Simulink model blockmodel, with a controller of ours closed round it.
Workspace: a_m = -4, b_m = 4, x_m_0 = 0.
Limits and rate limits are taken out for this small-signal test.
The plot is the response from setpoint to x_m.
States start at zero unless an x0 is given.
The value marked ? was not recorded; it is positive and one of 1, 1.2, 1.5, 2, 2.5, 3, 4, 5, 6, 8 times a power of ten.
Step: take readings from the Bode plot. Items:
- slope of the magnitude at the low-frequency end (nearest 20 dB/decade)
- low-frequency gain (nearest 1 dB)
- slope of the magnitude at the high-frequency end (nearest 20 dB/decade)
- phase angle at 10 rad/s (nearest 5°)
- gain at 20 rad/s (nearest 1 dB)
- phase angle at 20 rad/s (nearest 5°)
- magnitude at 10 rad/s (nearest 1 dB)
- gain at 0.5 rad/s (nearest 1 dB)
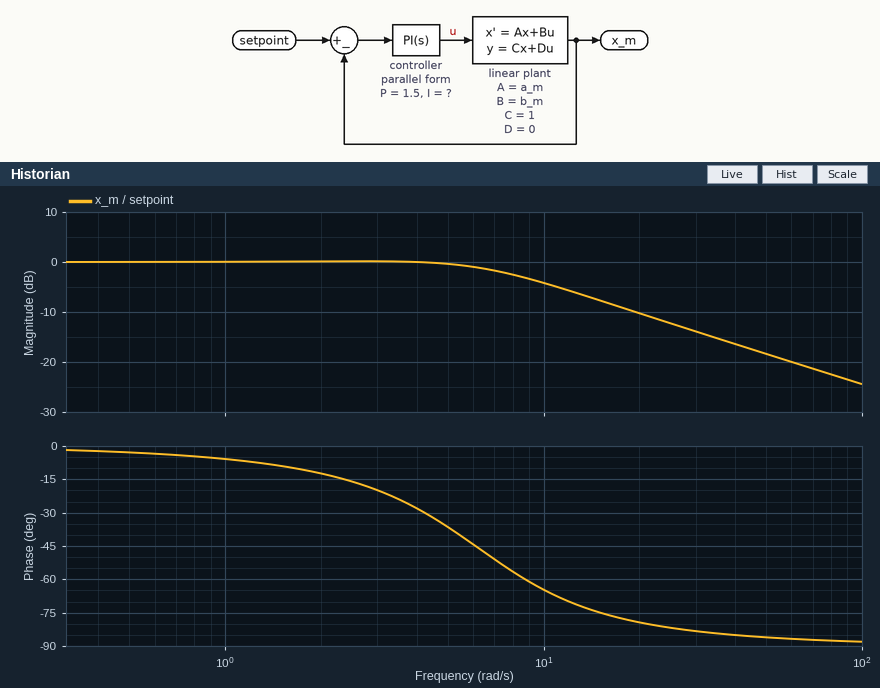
0 dB/decade
0 dB
-20 dB/decade
-65°
-10 dB
-80°
-4 dB
0 dB
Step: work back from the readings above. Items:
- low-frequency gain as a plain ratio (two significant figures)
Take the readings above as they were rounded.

1.0
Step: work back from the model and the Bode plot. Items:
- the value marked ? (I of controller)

10
